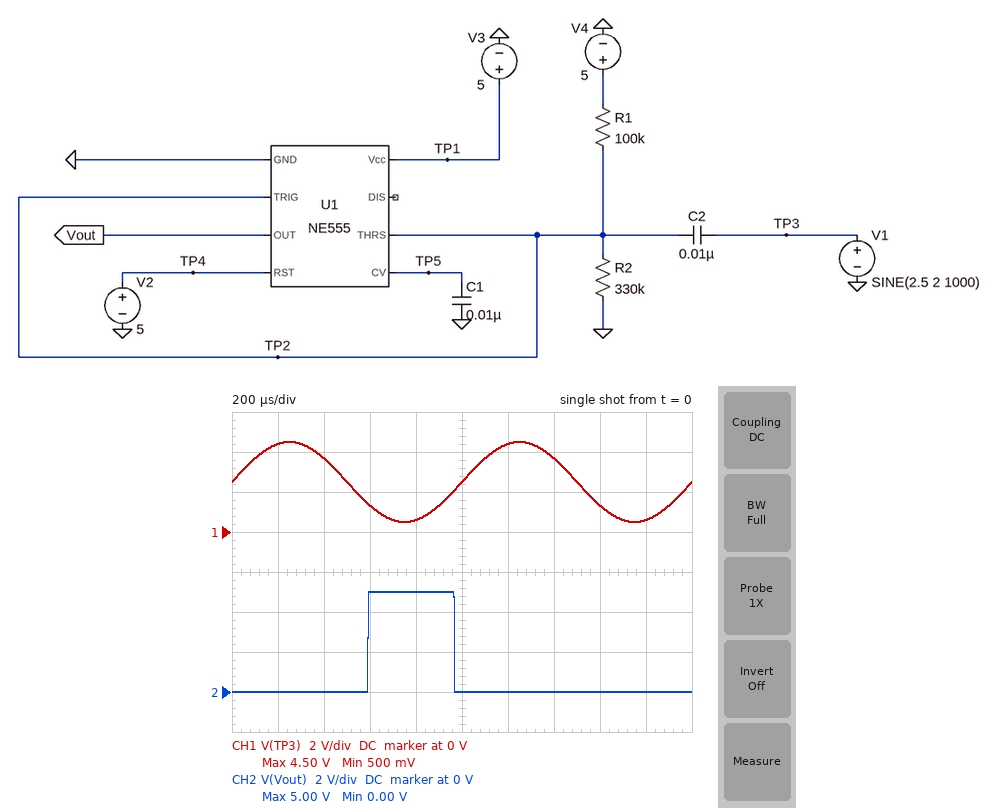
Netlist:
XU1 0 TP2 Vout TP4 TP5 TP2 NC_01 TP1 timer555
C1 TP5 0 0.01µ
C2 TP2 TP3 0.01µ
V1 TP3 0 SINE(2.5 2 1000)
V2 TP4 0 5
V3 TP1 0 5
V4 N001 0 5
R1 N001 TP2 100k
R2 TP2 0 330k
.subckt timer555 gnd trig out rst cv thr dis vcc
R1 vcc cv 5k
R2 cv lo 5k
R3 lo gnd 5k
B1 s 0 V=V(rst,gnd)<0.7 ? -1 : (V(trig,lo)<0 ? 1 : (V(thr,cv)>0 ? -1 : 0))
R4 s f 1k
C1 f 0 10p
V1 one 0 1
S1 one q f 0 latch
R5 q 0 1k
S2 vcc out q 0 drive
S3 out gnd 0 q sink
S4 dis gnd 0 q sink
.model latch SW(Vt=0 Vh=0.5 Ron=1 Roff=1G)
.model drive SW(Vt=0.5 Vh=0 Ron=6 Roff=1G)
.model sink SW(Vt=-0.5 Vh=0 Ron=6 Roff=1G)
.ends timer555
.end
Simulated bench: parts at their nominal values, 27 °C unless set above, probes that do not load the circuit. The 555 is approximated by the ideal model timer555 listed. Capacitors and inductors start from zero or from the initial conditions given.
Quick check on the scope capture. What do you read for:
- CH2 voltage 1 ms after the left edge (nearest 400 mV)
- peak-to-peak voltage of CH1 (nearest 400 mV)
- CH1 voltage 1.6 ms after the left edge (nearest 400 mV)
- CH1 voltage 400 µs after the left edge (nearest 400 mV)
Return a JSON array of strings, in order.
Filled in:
["0 V", "4.0 V", "1.2 V", "3.6 V"]
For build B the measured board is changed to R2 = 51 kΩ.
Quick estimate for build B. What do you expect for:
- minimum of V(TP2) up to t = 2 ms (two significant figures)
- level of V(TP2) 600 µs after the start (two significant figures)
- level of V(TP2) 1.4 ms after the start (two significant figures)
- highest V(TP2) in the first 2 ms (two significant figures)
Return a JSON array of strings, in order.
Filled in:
["-120 mV", "110 mV", "2.0 V", "3.5 V"]
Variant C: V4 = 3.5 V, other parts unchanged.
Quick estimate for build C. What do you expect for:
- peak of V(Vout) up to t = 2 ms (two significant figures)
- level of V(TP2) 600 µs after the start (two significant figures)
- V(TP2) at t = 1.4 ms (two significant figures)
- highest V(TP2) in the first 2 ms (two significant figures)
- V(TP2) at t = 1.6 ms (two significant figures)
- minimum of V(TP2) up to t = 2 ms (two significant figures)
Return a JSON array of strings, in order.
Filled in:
["5.0 V", "970 mV", "3.4 V", "4.5 V", "1.2 V", "500 mV"]
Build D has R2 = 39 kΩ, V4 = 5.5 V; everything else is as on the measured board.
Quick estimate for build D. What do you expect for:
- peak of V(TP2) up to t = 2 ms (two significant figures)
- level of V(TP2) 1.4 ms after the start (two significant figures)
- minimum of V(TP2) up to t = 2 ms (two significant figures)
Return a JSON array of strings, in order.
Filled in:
["3.3 V", "1.7 V", "-200 mV"]
